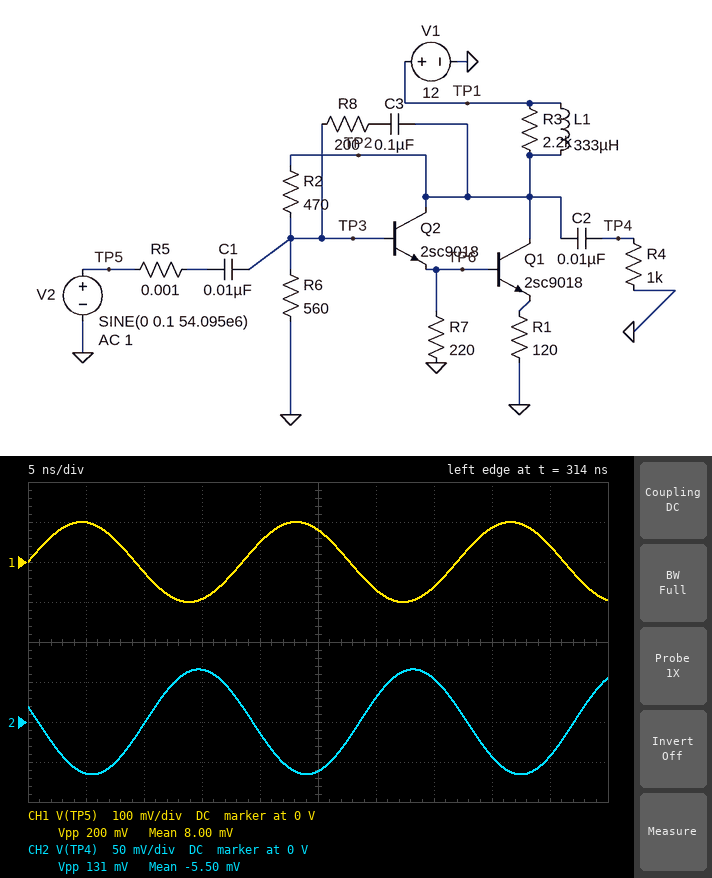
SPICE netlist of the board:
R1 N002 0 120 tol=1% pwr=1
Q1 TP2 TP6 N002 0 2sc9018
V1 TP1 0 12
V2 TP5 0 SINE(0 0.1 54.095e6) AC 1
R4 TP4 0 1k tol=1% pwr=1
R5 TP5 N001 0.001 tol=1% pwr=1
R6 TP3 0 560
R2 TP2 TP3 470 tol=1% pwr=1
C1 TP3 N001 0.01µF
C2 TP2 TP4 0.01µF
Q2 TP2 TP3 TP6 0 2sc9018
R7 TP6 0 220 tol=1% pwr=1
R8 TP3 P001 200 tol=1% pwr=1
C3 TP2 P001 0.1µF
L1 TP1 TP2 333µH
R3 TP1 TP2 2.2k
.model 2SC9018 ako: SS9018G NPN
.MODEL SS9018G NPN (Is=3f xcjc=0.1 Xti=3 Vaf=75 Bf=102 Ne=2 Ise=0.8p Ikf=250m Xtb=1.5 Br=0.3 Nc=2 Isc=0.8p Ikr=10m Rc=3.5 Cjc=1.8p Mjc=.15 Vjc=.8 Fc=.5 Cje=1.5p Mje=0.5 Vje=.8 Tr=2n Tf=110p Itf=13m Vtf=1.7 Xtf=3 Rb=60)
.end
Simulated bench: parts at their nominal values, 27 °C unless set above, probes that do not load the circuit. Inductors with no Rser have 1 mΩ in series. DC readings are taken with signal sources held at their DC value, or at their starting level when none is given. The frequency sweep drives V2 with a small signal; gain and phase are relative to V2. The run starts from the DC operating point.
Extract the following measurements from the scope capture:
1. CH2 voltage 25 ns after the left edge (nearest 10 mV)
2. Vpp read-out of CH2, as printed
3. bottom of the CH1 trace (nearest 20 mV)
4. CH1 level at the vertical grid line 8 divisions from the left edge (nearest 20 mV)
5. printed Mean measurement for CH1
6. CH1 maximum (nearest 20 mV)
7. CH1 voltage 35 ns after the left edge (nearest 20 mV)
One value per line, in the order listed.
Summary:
-60 mV
131 mV
-100 mV
80 mV
8.00 mV
100 mV
-60 mV
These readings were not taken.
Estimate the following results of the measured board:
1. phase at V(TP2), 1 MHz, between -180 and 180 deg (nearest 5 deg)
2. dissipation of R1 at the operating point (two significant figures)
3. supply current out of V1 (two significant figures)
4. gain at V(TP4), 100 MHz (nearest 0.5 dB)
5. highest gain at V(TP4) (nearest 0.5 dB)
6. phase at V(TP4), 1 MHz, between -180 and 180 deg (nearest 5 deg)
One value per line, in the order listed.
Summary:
-165 deg
200 mW
78 mA
-3.0 dB
2.0 dB
-165 deg
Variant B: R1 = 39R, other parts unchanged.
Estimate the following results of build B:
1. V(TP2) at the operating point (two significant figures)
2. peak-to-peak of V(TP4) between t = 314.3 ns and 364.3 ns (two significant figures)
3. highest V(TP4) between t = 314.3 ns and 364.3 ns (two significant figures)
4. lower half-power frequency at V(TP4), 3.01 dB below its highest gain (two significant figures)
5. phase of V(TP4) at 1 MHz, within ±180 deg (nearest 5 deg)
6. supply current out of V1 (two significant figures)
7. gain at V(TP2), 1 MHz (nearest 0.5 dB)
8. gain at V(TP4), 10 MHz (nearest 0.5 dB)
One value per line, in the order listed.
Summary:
12 V
500 mV
250 mV
470 kHz
-155 deg
160 mA
7.0 dB
8.0 dB
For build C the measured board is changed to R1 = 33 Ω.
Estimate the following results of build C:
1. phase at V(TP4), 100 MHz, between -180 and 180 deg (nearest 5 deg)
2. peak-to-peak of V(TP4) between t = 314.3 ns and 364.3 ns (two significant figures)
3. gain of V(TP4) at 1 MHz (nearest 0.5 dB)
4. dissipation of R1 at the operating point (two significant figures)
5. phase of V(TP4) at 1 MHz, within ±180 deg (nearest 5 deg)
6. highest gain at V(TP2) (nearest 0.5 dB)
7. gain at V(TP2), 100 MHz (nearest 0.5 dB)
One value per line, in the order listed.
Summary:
140 deg
590 mV
8.5 dB
680 mW
-150 deg
9.5 dB
9.0 dB
